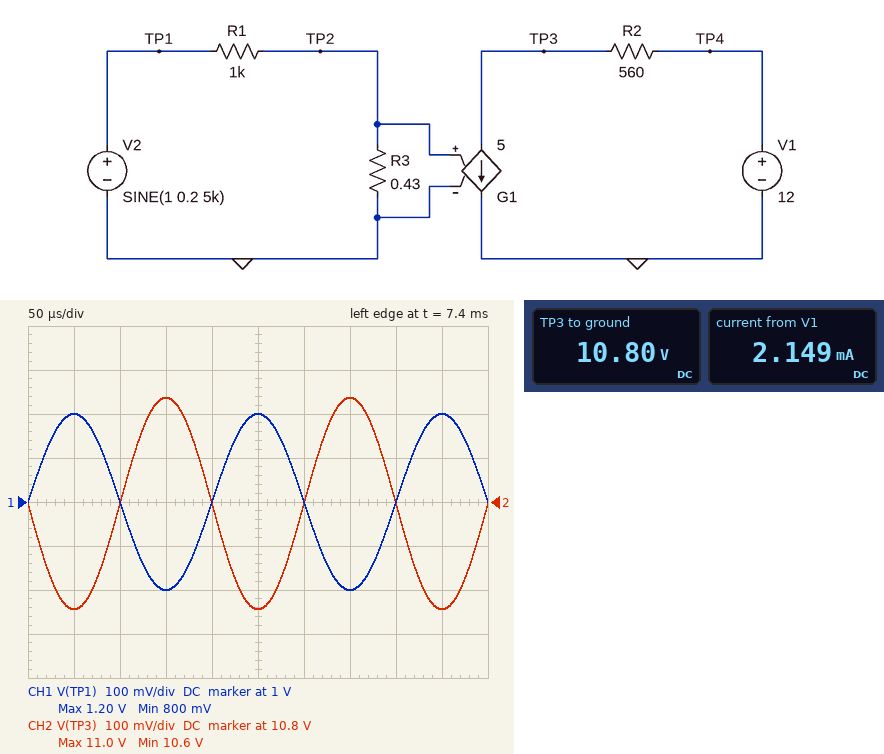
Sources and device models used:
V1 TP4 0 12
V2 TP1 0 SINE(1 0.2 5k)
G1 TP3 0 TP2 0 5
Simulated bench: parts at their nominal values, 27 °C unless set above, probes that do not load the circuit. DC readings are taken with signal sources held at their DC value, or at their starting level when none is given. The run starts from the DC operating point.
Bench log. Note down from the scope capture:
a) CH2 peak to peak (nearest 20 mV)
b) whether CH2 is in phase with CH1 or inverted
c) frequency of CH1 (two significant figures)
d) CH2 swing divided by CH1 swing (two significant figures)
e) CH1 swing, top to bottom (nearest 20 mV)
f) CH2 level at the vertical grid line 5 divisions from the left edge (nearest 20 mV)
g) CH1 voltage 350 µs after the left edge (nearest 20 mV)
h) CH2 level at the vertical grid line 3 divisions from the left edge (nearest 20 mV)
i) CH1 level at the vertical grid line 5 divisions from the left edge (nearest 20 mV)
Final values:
480 mV
inverted
5.0 kHz
1.2
400 mV
10.56 V
800 mV
11.04 V
1.20 V
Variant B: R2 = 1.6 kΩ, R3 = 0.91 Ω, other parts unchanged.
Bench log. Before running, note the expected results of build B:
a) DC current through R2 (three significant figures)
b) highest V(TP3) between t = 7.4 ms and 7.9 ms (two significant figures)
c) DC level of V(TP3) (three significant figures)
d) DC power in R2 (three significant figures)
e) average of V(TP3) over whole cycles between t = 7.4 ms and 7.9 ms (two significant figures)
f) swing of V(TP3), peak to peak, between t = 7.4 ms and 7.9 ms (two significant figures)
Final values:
4.55 mA
6.2 V
4.73 V
33.1 mW
4.7 V
2.9 V
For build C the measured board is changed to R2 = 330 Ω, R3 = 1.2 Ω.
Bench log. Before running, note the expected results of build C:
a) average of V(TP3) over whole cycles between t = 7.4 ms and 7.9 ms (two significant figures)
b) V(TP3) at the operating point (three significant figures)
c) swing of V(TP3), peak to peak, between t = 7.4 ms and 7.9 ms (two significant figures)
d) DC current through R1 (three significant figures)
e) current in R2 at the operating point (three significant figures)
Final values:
10 V
10.0 V
790 mV
999 µA
5.99 mA
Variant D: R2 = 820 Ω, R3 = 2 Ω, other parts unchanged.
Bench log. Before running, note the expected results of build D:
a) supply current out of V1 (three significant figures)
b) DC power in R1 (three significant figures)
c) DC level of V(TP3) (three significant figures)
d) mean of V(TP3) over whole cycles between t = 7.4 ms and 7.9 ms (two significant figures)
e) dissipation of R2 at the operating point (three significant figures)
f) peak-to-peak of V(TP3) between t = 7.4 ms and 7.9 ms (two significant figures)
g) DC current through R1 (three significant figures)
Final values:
9.98 mA
996 µW
3.82 V
3.8 V
81.7 mW
3.3 V
998 µA
